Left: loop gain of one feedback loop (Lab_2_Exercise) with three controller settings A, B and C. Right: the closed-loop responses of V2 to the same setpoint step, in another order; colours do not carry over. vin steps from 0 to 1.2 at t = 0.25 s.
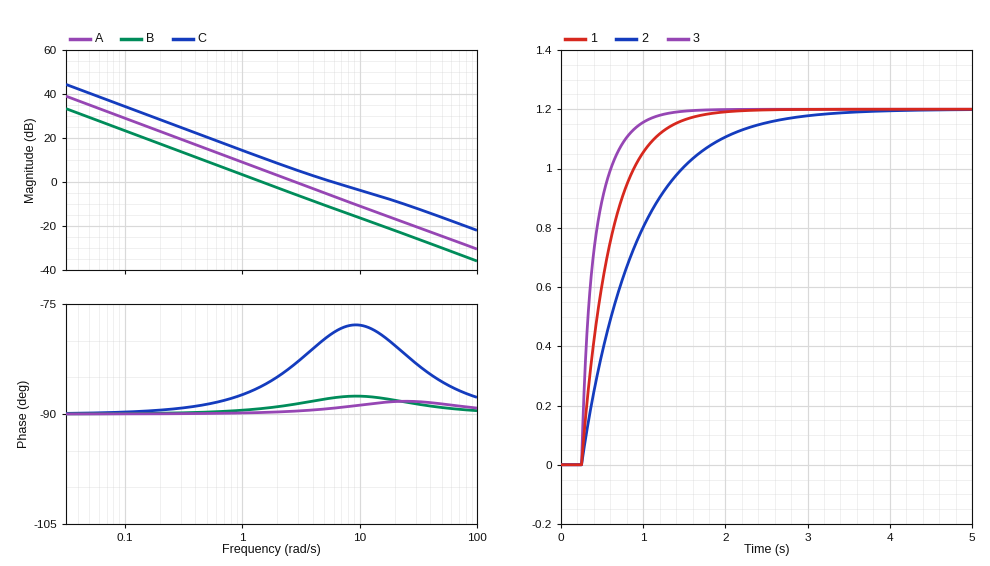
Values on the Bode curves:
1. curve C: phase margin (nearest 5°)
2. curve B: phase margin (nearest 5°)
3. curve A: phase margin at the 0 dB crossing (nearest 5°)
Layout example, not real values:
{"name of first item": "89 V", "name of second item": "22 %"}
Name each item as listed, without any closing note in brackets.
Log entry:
{"curve C: phase margin": "100°", "curve B: phase margin": "90°", "curve A: phase margin at the 0 dB crossing": "90°"}
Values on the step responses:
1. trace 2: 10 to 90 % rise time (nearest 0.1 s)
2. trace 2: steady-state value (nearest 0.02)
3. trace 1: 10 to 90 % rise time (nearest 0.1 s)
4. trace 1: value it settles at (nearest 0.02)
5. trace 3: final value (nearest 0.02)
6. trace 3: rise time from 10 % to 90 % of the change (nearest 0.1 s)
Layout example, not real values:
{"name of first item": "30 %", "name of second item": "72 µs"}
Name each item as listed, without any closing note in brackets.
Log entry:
{"trace 2: 10 to 90 % rise time": "1.5 s", "trace 2: steady-state value": "1.20", "trace 1: 10 to 90 % rise time": "0.8 s", "trace 1: value it settles at": "1.20", "trace 3: final value": "1.20", "trace 3: rise time from 10 % to 90 % of the change": "0.5 s"}
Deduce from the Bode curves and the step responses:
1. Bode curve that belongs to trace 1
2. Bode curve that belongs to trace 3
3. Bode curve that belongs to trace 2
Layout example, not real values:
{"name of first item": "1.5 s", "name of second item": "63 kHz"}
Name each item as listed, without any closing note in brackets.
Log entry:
{"Bode curve that belongs to trace 1": "A", "Bode curve that belongs to trace 3": "C", "Bode curve that belongs to trace 2": "B"}
